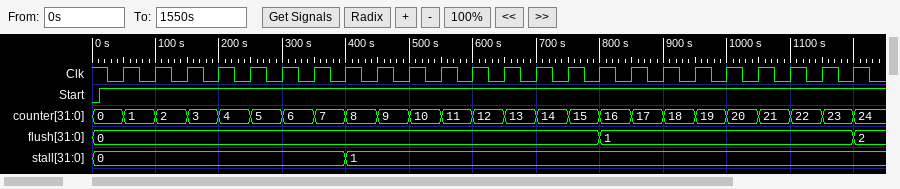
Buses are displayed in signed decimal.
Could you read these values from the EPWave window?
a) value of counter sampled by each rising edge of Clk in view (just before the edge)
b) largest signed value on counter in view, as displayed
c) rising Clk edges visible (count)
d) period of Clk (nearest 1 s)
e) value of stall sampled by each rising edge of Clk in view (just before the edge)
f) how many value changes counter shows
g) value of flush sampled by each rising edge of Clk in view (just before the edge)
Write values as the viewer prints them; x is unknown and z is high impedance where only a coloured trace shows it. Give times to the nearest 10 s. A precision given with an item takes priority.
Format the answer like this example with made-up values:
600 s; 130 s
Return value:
0, 1, 2, 3, 4, 5, 6, 7, 8, 9, 10, 11, 12, 13, 14, 15, 16, 17, 18, 19, 20, 21, 22, 23; 24; 24; 50 s; 0, 0, 0, 0, 0, 0, 0, 0, 1, 1, 1, 1, 1, 1, 1, 1, 1, 1, 1, 1, 1, 1, 1, 1; 24; 0, 0, 0, 0, 0, 0, 0, 0, 0, 0, 0, 0, 0, 0, 0, 0, 1, 1, 1, 1, 1, 1, 1, 1
